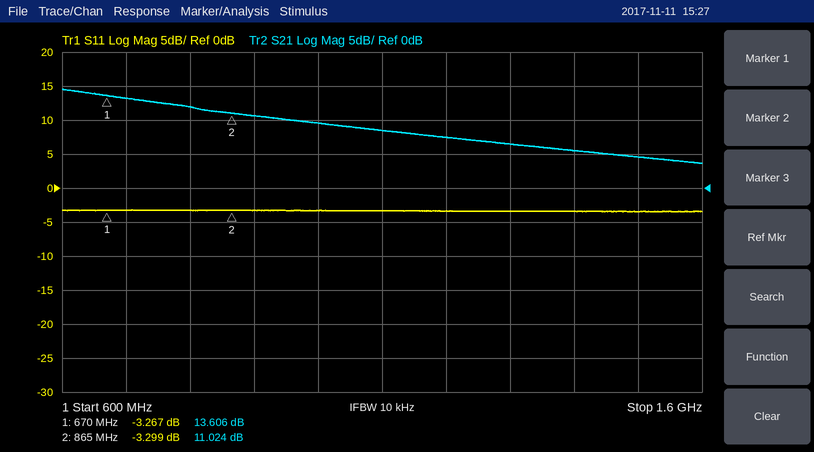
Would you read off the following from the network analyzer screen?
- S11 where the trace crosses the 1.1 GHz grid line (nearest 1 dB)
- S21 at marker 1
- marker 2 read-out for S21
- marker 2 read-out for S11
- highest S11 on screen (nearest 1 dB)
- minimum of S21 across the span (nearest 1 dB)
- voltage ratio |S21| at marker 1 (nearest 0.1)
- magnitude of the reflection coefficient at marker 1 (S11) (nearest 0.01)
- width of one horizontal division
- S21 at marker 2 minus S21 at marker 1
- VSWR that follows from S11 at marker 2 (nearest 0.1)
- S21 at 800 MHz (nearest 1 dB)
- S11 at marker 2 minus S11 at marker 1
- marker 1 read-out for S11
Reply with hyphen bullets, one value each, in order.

- -3 dB
- 13.606 dB
- 11.024 dB
- -3.299 dB
- -3 dB
- 4 dB
- 4.8
- 0.69
- 100 MHz
- -2.582 dB
- 5.3
- 12 dB
- -0.032 dB
- -3.267 dB
